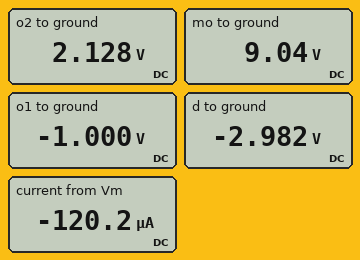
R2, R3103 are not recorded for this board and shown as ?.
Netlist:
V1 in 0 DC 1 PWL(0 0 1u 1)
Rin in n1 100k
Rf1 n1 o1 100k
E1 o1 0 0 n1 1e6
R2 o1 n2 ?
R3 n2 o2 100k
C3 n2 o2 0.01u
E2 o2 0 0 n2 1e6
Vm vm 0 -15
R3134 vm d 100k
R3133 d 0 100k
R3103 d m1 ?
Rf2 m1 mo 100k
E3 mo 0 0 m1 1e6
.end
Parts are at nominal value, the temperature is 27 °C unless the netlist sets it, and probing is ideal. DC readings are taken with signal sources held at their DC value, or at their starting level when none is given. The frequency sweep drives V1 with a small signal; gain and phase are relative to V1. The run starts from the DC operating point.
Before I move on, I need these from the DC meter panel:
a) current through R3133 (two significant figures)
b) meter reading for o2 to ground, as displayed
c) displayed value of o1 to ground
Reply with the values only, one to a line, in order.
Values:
30 µA
2.128 V
-1.000 V
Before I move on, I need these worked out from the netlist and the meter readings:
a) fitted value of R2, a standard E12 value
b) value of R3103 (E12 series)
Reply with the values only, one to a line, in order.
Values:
47 kΩ
33 kΩ
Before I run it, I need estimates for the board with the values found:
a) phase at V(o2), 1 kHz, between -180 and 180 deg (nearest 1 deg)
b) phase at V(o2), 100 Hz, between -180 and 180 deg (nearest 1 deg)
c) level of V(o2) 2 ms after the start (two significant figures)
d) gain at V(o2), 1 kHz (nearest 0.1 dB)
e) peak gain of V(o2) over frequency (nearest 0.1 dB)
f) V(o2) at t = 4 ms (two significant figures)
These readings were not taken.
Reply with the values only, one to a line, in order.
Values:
-81 deg
-32 deg
1.8 V
-9.5 dB
6.6 dB
2.1 V
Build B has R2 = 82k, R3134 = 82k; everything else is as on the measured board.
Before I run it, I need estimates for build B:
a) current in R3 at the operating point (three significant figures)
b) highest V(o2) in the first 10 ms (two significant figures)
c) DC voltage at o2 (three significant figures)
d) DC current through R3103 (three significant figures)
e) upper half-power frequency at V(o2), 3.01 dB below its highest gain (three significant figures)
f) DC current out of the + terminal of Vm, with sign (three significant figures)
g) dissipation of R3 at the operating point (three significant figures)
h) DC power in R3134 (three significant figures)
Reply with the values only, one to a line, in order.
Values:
12.2 µA
1.2 V
1.22 V
106 µA
159 Hz
-140 µA
14.9 µW
1.62 mW
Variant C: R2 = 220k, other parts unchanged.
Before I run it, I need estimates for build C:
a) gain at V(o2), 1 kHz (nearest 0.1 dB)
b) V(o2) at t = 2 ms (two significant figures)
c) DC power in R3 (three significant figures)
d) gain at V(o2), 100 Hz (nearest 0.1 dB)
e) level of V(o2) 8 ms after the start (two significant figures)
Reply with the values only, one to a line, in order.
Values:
-22.9 dB
390 mV
2.07 µW
-8.3 dB
450 mV
